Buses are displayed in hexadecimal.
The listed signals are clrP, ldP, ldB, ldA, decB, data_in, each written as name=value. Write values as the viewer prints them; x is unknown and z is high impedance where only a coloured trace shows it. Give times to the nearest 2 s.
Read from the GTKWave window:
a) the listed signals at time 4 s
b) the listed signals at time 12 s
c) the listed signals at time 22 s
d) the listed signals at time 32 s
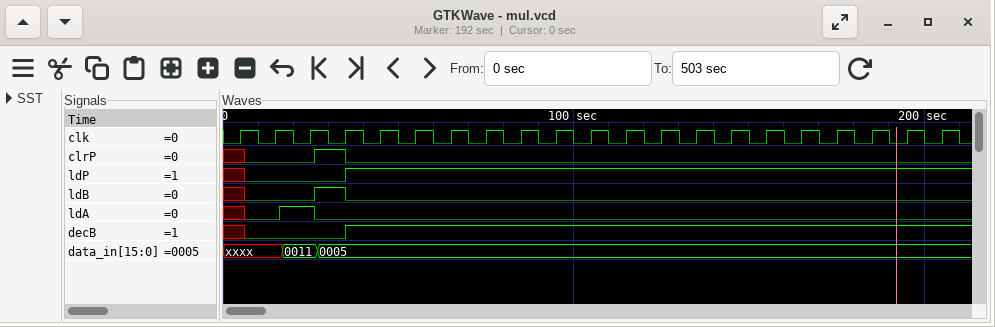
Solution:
clrP=x, ldP=x, ldB=x, ldA=x, decB=x, data_in=xxxx
clrP=0, ldP=0, ldB=0, ldA=0, decB=0, data_in=xxxx
clrP=0, ldP=0, ldB=0, ldA=1, decB=0, data_in=0011
clrP=1, ldP=0, ldB=1, ldA=0, decB=0, data_in=0005
